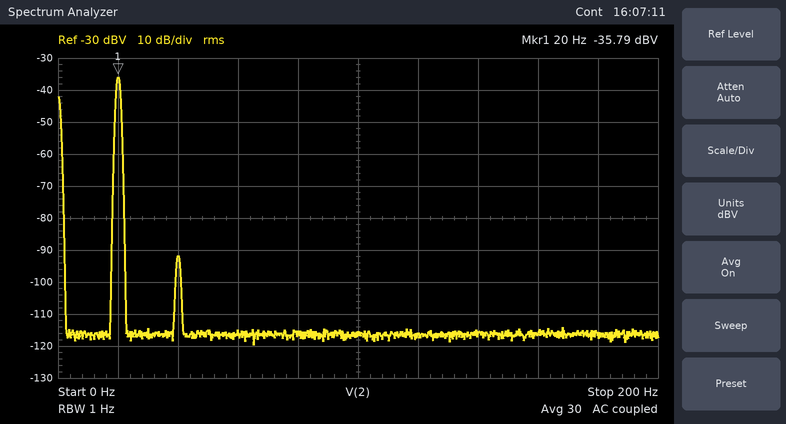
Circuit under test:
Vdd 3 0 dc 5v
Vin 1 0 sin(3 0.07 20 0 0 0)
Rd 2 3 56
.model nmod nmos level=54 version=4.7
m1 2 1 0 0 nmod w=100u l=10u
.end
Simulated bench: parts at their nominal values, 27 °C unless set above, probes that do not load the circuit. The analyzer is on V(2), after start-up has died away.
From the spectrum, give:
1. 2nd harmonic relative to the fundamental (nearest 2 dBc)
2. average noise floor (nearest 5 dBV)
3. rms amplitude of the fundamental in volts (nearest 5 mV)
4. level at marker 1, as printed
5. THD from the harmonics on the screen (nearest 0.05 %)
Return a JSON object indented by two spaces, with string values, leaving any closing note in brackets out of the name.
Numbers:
{
  "2nd harmonic relative to the fundamental": "-56 dBc",
  "average noise floor": "-115 dBV",
  "rms amplitude of the fundamental in volts": "15 mV",
  "level at marker 1, as printed": "-35.79 dBV",
  "THD from the harmonics on the screen": "0.15 %"
}
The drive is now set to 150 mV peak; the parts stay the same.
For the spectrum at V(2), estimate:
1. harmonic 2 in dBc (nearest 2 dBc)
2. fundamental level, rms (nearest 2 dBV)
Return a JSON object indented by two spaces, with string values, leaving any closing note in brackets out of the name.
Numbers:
{
  "harmonic 2 in dBc": "-50 dBc",
  "fundamental level, rms": "-30 dBV"
}
